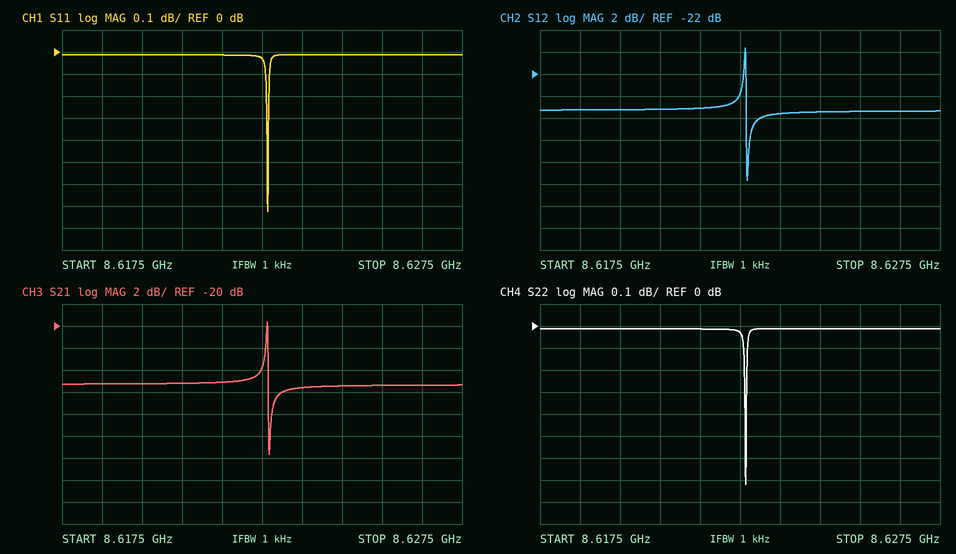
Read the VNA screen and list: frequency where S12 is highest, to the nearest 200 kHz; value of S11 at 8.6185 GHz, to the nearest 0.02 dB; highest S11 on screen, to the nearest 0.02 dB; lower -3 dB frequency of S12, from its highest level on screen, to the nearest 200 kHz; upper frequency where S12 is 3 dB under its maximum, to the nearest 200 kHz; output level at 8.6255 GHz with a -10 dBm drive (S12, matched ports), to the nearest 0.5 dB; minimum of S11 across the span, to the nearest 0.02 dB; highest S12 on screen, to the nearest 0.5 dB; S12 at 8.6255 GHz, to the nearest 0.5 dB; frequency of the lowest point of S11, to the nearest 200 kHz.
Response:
8.6226 GHz
-0.02 dB
-0.02 dB
8.6226 GHz
8.6226 GHz
-35.5 dBm
-0.72 dB
-19.5 dB
-25.5 dB
8.6226 GHz
